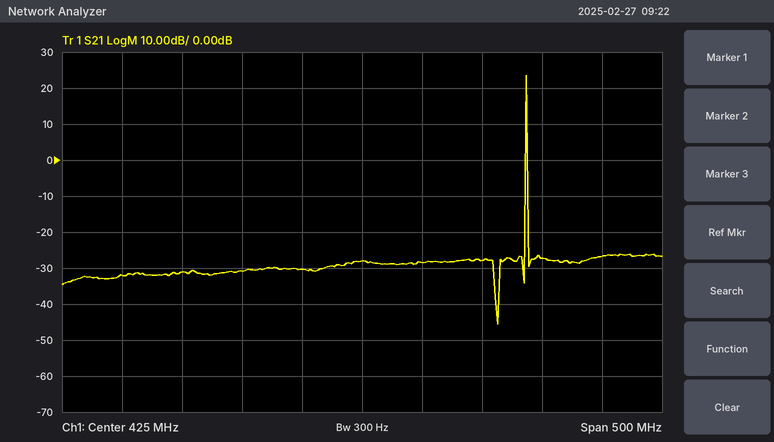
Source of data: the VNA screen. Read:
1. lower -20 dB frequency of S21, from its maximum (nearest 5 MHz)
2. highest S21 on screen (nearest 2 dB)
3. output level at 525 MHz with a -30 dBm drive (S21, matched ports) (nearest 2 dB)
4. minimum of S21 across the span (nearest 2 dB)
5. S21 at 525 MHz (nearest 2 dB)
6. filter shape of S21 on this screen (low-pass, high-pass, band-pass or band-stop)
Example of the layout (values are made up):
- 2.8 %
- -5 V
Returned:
- 560 MHz
- 24 dB
- -58 dBm
- -46 dB
- -28 dB
- band-pass
